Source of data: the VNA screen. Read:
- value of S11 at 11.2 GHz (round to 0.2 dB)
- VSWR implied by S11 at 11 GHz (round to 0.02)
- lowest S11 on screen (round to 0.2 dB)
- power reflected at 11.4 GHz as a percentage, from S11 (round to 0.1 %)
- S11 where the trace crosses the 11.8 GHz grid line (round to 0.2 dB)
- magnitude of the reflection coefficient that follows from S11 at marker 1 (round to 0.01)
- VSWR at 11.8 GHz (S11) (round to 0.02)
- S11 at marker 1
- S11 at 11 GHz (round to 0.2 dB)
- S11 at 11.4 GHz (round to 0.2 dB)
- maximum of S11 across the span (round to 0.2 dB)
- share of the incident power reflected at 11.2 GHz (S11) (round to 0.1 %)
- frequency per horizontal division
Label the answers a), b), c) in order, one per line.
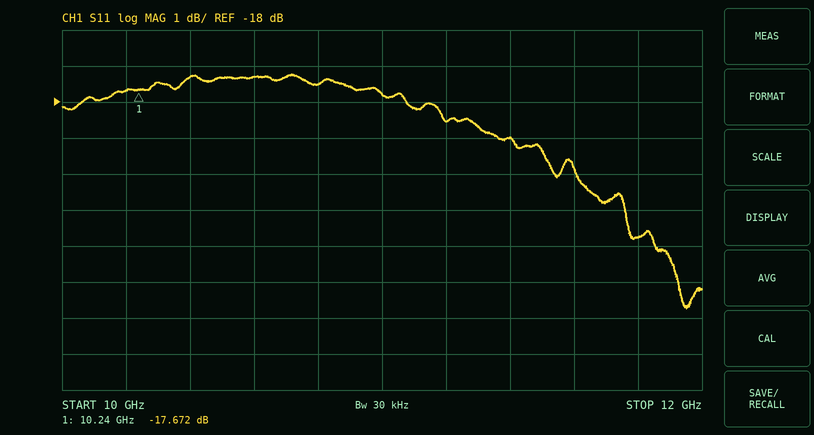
a) -18.6 dB
b) 1.30
c) -23.8 dB
d) 1.3 %
e) -21.8 dB
f) 0.13
g) 1.18
h) -17.672 dB
i) -17.8 dB
j) -19.0 dB
k) -17.2 dB
l) 1.4 %
m) 200 MHz
